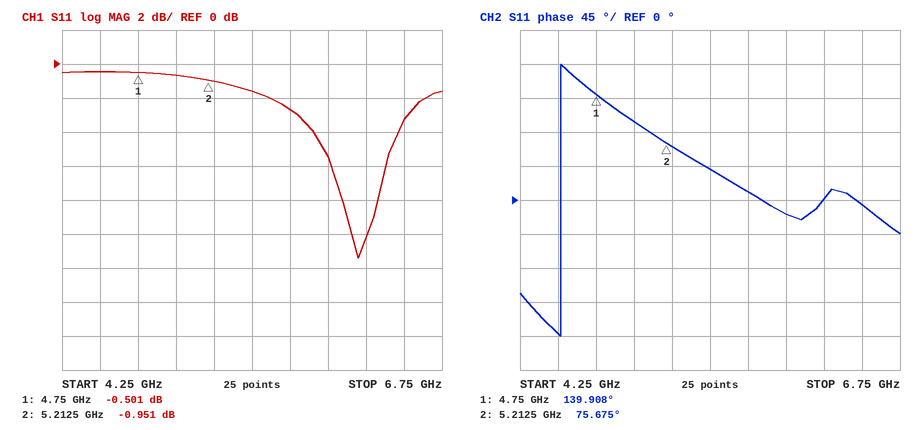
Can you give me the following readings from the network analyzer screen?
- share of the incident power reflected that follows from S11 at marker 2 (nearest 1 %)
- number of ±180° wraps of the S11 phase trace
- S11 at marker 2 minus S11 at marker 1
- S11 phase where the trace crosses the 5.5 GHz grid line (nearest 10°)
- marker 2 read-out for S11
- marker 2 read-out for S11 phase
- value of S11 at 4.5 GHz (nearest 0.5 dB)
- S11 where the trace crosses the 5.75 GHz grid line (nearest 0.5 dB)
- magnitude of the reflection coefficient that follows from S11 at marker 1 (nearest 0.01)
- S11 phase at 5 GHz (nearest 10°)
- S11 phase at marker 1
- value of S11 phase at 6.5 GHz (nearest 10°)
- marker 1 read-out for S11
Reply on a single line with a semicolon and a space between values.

80 %; 1; -0.450 dB; 40°; -0.951 dB; 75.675°; -0.5 dB; -2.5 dB; 0.94; 100°; 139.908°; -10°; -0.501 dB
